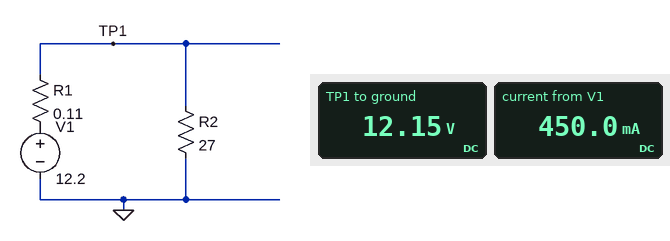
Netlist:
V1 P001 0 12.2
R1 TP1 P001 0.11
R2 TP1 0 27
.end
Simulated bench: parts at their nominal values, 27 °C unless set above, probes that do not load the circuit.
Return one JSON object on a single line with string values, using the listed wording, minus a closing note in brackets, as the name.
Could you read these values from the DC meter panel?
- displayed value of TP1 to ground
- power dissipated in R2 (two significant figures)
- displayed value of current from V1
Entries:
{"displayed value of TP1 to ground": "12.15 V", "power dissipated in R2": "5.5 W", "displayed value of current from V1": "450.0 mA"}
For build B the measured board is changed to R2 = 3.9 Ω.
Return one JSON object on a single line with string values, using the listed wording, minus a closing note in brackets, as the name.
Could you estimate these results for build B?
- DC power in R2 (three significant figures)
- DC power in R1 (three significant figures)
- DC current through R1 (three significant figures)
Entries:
{"DC power in R2": "36.1 W", "DC power in R1": "1.02 W", "DC current through R1": "3.04 A"}
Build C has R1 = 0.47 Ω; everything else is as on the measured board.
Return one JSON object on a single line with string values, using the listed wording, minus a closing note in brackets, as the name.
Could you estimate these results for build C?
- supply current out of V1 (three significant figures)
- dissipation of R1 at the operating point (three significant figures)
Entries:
{"supply current out of V1": "444 mA", "dissipation of R1 at the operating point": "92.7 mW"}
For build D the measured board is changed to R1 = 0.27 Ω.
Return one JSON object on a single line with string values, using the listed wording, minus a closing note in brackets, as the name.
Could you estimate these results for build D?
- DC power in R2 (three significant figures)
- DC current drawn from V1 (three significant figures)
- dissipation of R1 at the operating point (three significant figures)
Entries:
{"DC power in R2": "5.40 W", "DC current drawn from V1": "447 mA", "dissipation of R1 at the operating point": "54.0 mW"}
